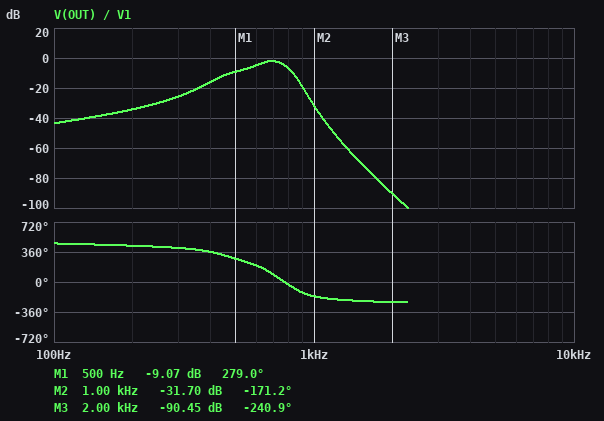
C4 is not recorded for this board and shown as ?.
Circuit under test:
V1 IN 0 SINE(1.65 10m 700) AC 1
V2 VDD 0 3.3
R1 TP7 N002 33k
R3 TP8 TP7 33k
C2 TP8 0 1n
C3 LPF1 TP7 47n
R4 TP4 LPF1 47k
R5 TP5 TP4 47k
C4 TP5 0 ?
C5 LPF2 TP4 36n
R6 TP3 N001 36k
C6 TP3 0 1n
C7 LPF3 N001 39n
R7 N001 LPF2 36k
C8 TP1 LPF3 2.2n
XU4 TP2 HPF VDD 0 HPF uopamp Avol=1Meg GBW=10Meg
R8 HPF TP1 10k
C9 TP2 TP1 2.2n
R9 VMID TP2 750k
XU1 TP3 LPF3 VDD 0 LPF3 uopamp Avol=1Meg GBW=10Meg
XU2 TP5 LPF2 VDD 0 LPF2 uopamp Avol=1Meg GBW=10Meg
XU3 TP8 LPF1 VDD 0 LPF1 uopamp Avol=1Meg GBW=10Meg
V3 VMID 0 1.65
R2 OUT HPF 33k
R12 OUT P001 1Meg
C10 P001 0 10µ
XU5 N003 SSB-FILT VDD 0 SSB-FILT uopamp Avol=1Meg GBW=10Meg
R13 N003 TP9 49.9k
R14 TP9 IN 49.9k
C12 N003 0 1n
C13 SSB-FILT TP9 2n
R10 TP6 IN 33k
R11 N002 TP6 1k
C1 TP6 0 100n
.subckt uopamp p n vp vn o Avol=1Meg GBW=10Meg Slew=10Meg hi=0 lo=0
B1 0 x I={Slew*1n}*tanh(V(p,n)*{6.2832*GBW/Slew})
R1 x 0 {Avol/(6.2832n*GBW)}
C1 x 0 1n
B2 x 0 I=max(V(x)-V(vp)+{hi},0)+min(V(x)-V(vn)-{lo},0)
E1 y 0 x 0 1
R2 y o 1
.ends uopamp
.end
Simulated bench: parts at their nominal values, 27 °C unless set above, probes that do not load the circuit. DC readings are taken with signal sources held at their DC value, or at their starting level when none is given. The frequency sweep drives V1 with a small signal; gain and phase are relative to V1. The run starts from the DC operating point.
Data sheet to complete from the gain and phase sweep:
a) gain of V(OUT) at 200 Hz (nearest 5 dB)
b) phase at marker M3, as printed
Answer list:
-35 dB
-240.9 deg
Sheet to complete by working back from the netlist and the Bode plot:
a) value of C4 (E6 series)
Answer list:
1.5 nF
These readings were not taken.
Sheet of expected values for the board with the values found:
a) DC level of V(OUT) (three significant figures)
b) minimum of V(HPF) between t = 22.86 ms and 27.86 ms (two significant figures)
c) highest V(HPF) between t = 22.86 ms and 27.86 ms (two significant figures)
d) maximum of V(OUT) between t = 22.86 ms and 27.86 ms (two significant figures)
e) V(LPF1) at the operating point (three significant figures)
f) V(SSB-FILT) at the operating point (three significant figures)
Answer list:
1.65 V
1.6 V
1.7 V
1.7 V
1.65 V
1.65 V
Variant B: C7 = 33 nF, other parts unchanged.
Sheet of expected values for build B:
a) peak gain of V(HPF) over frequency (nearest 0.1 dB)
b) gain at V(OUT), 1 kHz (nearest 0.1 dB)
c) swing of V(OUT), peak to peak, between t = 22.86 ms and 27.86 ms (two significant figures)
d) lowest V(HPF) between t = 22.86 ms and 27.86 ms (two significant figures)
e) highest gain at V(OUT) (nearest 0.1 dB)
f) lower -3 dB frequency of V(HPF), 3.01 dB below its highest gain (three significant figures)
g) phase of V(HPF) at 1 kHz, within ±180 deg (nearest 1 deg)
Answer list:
-2.7 dB
-29.2 dB
14 mV
1.6 V
-3.0 dB
615 Hz
-162 deg
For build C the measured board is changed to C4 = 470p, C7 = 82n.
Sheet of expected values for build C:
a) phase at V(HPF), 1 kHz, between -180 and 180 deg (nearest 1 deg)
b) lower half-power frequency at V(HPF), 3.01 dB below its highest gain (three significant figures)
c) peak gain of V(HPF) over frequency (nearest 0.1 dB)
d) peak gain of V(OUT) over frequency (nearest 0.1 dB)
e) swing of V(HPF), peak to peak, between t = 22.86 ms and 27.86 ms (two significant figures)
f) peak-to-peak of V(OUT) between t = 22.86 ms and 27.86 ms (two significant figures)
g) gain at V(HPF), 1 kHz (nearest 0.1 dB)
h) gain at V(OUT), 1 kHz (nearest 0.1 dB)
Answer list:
-171 deg
649 Hz
1.4 dB
1.1 dB
20 mV
19 mV
-24.0 dB
-24.3 dB
